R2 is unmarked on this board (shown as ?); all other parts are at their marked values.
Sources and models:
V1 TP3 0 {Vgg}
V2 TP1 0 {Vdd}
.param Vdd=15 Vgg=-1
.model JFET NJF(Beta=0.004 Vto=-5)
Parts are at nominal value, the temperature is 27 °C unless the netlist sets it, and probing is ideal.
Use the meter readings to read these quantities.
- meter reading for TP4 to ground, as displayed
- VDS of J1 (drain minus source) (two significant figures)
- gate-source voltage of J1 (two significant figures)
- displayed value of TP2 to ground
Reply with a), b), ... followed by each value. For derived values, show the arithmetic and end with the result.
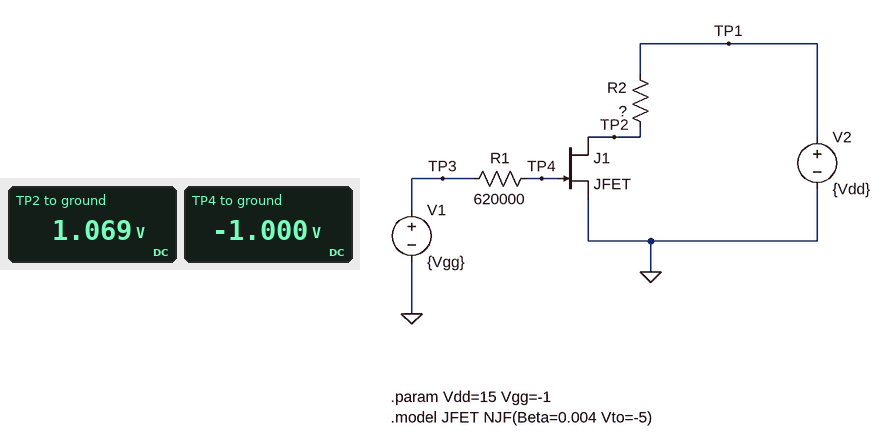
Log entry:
a) -1.000 V
b) 1.069 V = 1.1 V
c) -1 V = -1.0 V
d) 1.069 V
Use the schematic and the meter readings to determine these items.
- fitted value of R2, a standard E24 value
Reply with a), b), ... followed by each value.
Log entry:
a) 470 Ω
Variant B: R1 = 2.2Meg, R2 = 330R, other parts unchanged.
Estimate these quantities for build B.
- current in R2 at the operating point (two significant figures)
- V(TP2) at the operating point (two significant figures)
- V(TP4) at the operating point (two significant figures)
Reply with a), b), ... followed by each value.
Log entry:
a) 41 mA
b) 1.6 V
c) -1.0 V
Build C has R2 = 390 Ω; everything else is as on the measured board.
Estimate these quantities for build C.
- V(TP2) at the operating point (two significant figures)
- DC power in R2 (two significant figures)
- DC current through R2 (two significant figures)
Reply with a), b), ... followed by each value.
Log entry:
a) 1.3 V
b) 480 mW
c) 35 mA
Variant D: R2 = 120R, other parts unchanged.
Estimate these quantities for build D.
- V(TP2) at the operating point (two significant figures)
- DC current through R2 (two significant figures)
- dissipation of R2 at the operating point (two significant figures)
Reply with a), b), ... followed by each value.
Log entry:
a) 7.3 V
b) 64 mA
c) 490 mW
